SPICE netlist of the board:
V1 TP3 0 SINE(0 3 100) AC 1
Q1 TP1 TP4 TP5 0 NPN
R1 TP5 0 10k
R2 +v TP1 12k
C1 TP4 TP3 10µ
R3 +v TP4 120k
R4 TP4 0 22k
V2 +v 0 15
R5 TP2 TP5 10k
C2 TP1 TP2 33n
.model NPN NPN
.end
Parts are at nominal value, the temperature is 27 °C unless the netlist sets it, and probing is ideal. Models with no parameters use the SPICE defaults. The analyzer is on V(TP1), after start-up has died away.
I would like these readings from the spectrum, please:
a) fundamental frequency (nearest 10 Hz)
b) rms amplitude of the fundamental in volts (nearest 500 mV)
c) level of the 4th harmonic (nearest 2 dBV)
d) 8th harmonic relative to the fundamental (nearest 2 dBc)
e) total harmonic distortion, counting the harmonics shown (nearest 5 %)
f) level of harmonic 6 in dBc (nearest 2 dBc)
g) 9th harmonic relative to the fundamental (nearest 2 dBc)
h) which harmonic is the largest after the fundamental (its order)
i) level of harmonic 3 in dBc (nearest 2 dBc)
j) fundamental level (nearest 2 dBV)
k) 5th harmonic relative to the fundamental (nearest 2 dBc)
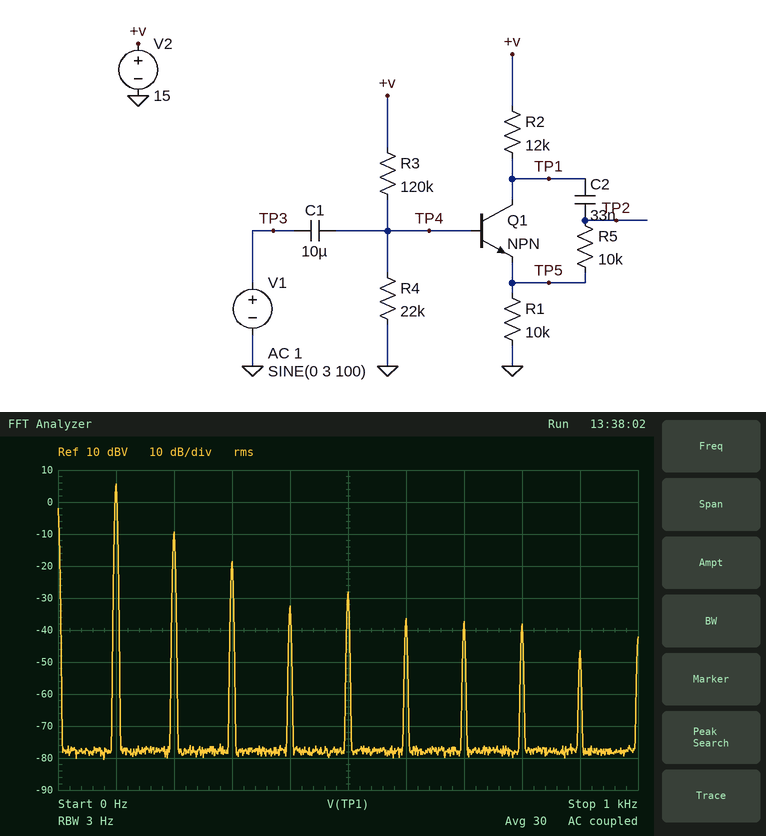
100 Hz
2.0 V
-32 dBV
-44 dBc
20 %
-42 dBc
-52 dBc
2
-24 dBc
6 dBV
-34 dBc
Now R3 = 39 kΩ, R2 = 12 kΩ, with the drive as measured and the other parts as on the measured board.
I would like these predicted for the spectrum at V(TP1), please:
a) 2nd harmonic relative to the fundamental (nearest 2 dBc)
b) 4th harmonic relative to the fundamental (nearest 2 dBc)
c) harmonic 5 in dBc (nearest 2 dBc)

-22 dBc
-26 dBc
-30 dBc
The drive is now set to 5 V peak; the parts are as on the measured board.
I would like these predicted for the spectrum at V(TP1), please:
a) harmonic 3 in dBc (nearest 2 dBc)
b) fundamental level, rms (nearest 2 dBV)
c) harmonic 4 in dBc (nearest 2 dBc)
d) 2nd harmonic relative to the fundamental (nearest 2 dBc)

-26 dBc
8 dBV
-28 dBc
-12 dBc
